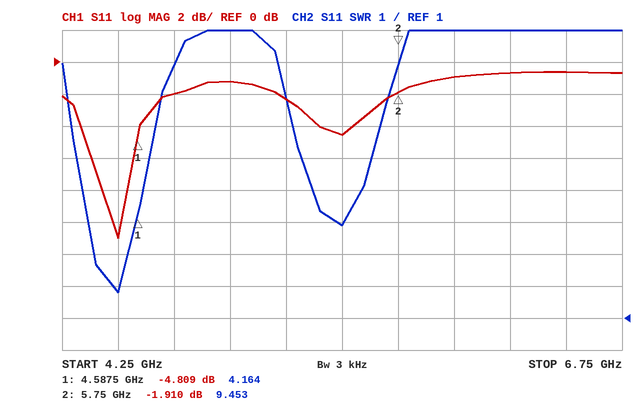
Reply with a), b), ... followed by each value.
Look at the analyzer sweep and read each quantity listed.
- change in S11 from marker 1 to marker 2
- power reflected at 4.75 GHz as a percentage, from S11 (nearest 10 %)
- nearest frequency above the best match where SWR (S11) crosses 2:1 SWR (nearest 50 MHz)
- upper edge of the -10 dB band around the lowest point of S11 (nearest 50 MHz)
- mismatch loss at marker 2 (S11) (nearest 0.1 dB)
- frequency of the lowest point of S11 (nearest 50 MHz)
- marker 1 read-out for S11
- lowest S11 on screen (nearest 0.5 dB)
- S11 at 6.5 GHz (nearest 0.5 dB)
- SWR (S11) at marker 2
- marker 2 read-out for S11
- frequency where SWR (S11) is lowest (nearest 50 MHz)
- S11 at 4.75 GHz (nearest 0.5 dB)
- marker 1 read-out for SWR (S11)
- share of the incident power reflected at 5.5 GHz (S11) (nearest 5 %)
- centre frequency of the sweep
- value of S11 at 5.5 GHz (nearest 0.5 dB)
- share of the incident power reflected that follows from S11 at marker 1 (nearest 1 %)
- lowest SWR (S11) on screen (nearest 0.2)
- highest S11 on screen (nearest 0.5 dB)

a) 2.899 dB
b) 60 %
c) 4.50 GHz
d) 4.50 GHz
e) 4.5 dB
f) 4.50 GHz
g) -4.809 dB
h) -11.0 dB
i) -0.5 dB
j) 9.453
k) -1.910 dB
l) 4.50 GHz
m) -2.0 dB
n) 4.164
o) 35 %
p) 5.5 GHz
q) -4.5 dB
r) 33 %
s) 1.8
t) -0.5 dB
